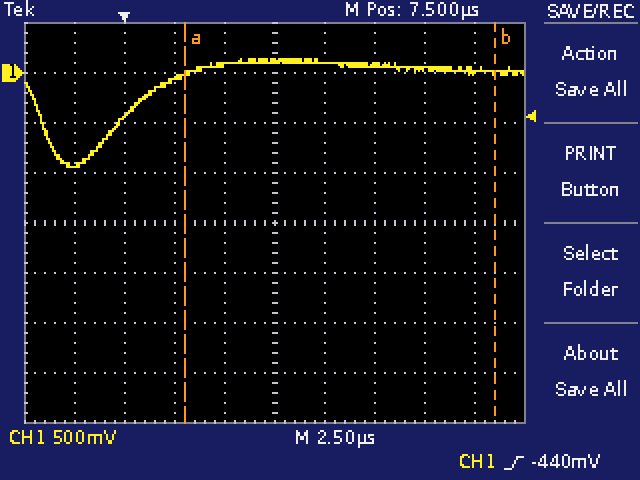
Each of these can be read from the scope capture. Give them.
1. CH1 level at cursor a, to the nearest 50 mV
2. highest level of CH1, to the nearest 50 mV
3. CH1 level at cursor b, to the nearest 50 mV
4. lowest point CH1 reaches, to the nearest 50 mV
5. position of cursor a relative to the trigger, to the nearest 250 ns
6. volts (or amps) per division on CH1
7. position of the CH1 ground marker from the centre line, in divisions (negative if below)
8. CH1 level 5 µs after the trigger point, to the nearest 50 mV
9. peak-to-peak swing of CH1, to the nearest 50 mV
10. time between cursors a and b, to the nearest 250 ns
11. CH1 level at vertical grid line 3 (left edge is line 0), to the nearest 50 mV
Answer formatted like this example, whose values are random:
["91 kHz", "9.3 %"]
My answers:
["0 mV", "150 mV", "0 mV", "-950 mV", "+3.00 µs", "500 mV", "+3.0 div", "100 mV", "1.10 V", "15.50 µs", "-50 mV"]
